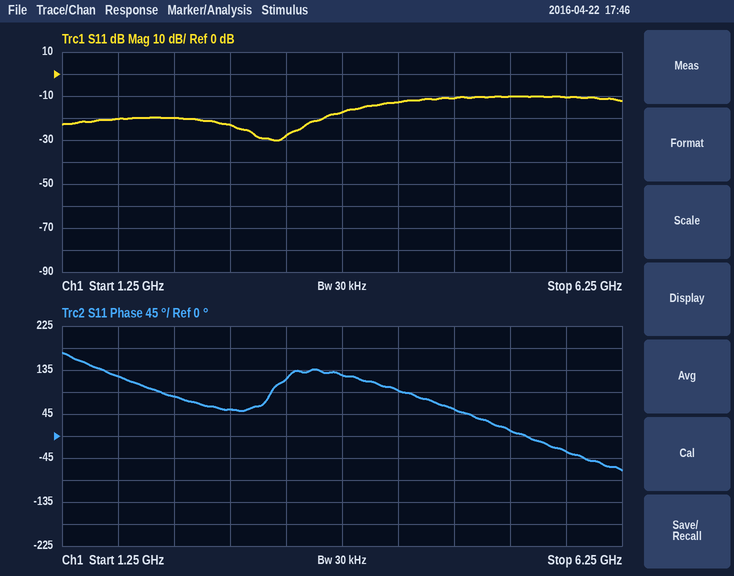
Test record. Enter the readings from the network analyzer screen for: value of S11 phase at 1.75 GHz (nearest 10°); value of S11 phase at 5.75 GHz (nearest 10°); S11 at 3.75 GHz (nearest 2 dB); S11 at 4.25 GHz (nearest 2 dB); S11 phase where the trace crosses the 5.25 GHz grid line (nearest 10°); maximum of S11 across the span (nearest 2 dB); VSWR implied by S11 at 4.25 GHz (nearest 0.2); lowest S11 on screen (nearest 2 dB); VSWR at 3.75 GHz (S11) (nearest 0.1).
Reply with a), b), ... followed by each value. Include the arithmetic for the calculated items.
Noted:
a) 120°
b) -30°
c) -18 dB
d) -12 dB
e) 10°
f) -10 dB
g) |Γ| = 10^(-12/20) = 0.2512; VSWR = (1 + 0.2512)/(1 − 0.2512) ≈ 1.67, so 1.6 to the nearest 0.2
h) -30 dB
i) |Γ| = 10^(-18/20) = 0.1259; VSWR = (1 + 0.1259)/(1 − 0.1259) ≈ 1.3
